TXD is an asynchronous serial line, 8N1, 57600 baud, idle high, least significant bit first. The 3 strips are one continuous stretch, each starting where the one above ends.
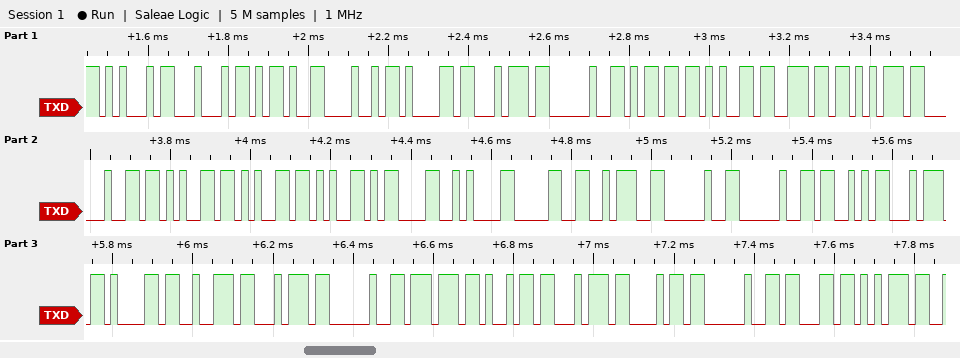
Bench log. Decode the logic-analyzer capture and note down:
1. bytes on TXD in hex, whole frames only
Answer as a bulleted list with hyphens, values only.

- 0x45 0x44 0x2D 0x48 0x61 0x74 0x20 0x6D 0x65 0x6E 0x75 0x20 0x2B 0x2B 0x2B 0x0D 0x0A 0x30 0x3A 0x20 0x20 0x53 0x74 0x61 0x72 0x74 0x20 0x77 0x69 0x74 0x68 0x20 0x63 0x75
